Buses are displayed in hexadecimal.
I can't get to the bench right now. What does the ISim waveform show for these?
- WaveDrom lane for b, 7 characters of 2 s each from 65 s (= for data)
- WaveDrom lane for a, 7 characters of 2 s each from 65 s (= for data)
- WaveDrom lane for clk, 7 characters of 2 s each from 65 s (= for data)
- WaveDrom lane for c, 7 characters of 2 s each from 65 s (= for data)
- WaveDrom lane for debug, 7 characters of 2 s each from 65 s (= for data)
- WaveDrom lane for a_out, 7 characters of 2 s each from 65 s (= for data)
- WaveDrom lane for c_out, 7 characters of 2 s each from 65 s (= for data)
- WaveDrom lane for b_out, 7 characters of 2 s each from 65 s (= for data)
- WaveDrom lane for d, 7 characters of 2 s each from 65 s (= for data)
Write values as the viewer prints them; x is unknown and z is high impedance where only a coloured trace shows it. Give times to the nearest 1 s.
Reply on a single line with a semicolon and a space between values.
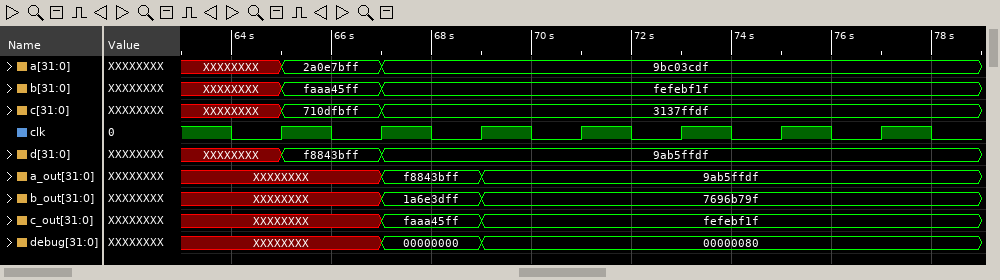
{name: 'b', wave: '==.....', data: 'faaa45ff fefebf1f'}; {name: 'a', wave: '==.....', data: '2a0e7bff 9bc03cdf'}; {name: 'clk', wave: 'p......'}; {name: 'c', wave: '==.....', data: '710dfbff 3137ffdf'}; {name: 'debug', wave: 'x==....', data: '00000000 00000080'}; {name: 'a_out', wave: 'x==....', data: 'f8843bff 9ab5ffdf'}; {name: 'c_out', wave: 'x==....', data: 'faaa45ff fefebf1f'}; {name: 'b_out', wave: 'x==....', data: '1a6e3dff 7696b79f'}; {name: 'd', wave: '==.....', data: 'f8843bff 9ab5ffdf'}
